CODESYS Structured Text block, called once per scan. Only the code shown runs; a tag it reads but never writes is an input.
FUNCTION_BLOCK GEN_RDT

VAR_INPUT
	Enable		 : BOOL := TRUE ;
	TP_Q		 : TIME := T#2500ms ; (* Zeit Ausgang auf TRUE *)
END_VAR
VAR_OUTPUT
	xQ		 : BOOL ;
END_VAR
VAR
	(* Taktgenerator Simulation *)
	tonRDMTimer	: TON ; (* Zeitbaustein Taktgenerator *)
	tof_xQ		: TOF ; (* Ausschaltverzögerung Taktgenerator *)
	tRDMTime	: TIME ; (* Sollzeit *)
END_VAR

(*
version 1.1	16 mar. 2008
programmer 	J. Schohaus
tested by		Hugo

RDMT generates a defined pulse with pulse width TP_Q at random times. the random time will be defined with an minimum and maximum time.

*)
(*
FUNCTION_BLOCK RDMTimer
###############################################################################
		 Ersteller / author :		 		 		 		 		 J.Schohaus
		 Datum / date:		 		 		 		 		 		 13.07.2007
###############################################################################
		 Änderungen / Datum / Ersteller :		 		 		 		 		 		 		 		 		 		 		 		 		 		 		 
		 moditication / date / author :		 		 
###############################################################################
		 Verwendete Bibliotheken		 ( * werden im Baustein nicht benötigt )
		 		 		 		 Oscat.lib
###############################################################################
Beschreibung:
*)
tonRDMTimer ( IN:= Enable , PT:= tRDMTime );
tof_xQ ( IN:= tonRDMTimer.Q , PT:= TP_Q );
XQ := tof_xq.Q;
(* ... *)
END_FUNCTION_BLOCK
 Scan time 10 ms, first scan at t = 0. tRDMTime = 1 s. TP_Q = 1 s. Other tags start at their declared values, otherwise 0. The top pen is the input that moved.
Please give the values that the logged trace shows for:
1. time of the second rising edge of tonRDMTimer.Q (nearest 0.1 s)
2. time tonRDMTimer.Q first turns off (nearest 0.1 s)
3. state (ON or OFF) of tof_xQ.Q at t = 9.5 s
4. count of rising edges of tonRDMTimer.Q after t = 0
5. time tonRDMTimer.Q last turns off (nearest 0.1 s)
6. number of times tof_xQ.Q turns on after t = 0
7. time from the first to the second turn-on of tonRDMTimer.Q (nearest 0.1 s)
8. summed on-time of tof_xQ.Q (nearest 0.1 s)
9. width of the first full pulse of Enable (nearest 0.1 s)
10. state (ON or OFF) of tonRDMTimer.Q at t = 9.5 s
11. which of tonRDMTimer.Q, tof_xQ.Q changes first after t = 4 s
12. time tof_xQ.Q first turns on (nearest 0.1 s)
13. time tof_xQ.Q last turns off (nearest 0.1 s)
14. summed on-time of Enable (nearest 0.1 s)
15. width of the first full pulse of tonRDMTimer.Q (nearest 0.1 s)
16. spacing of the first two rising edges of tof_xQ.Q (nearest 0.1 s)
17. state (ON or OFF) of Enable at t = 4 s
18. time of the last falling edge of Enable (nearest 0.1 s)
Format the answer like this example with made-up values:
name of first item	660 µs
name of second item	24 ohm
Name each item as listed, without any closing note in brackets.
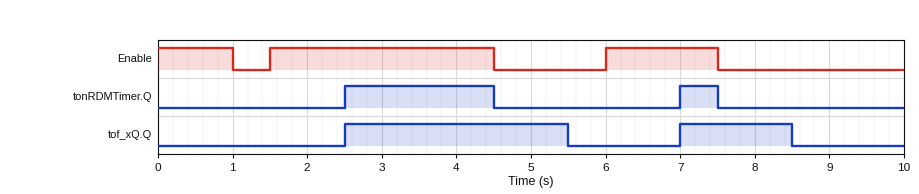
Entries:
time of the second rising edge of tonRDMTimer.Q	7.0 s
time tonRDMTimer.Q first turns off	4.5 s
state (ON or OFF) of tof_xQ.Q at t = 9.5 s	OFF
count of rising edges of tonRDMTimer.Q after t = 0	2
time tonRDMTimer.Q last turns off	7.5 s
number of times tof_xQ.Q turns on after t = 0	2
time from the first to the second turn-on of tonRDMTimer.Q	4.5 s
summed on-time of tof_xQ.Q	4.5 s
width of the first full pulse of Enable	3.0 s
state (ON or OFF) of tonRDMTimer.Q at t = 9.5 s	OFF
which of tonRDMTimer.Q, tof_xQ.Q changes first after t = 4 s	tonRDMTimer.Q
time tof_xQ.Q first turns on	2.5 s
time tof_xQ.Q last turns off	8.5 s
summed on-time of Enable	5.5 s
width of the first full pulse of tonRDMTimer.Q	2.0 s
spacing of the first two rising edges of tof_xQ.Q	4.5 s
state (ON or OFF) of Enable at t = 4 s	ON
time of the last falling edge of Enable	7.5 s
